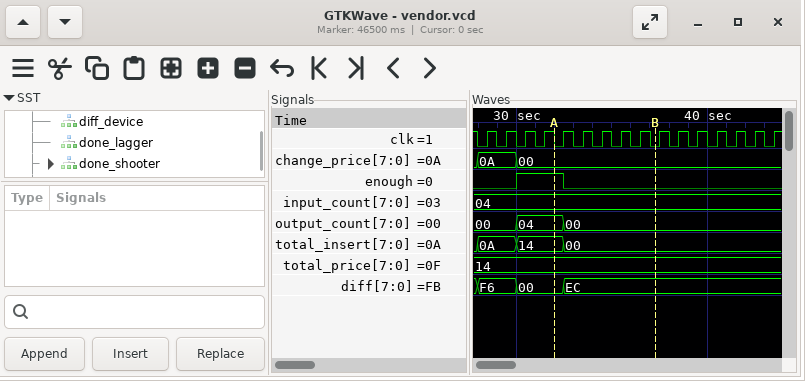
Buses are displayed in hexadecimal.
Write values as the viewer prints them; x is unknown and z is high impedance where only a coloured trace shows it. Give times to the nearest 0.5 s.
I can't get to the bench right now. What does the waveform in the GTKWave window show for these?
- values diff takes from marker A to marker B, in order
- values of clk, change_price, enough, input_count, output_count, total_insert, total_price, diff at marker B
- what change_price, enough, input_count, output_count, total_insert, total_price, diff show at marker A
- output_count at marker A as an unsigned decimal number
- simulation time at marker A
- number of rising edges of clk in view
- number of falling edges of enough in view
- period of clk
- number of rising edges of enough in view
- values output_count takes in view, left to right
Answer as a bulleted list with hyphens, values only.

- 00, EC
- clk=0, change_price=00, enough=0, input_count=04, output_count=00, total_insert=00, total_price=14, diff=EC
- change_price=00, enough=1, input_count=04, output_count=04, total_insert=14, total_price=14, diff=00
- 4
- 32 s
- 16
- 1
- 1 s
- 1
- 00, 04, 00
